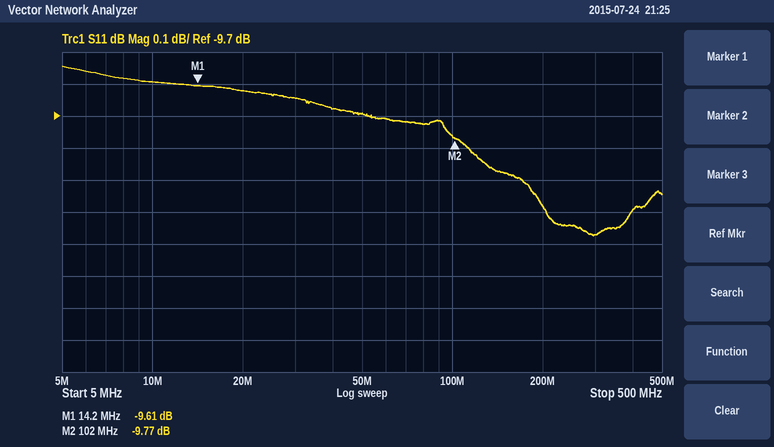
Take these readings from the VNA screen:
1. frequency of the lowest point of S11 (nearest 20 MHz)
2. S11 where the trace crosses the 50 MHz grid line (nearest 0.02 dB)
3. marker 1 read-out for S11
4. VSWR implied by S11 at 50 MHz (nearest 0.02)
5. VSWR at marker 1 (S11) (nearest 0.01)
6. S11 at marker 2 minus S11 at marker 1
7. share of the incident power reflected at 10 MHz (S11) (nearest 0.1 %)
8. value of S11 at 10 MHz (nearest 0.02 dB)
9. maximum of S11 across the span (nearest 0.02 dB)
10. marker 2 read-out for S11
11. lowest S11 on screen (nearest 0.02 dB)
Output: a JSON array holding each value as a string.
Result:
["300 MHz", "-9.70 dB", "-9.61 dB", "1.98", "1.99", "-0.16 dB", "11.0 %", "-9.60 dB", "-9.54 dB", "-9.77 dB", "-10.08 dB"]
